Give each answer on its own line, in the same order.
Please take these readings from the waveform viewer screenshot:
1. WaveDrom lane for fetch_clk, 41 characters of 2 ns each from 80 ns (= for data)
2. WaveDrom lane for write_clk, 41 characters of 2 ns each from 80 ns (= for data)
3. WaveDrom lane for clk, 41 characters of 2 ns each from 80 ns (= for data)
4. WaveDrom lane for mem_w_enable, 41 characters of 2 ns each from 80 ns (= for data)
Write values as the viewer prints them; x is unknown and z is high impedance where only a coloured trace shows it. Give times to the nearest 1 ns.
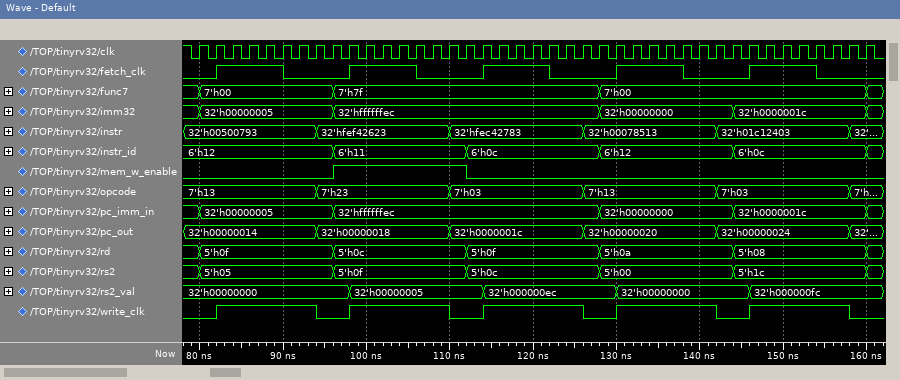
{name: 'fetch_clk', wave: '01...0...1...0...1...0...1...0...1...0...'}
{name: 'write_clk', wave: '01.....0.1.....0.1.....0.1.....0.1.....0.'}
{name: 'clk', wave: 'p........................................'}
{name: 'mem_w_enable', wave: '0.......1.......0........................'}
